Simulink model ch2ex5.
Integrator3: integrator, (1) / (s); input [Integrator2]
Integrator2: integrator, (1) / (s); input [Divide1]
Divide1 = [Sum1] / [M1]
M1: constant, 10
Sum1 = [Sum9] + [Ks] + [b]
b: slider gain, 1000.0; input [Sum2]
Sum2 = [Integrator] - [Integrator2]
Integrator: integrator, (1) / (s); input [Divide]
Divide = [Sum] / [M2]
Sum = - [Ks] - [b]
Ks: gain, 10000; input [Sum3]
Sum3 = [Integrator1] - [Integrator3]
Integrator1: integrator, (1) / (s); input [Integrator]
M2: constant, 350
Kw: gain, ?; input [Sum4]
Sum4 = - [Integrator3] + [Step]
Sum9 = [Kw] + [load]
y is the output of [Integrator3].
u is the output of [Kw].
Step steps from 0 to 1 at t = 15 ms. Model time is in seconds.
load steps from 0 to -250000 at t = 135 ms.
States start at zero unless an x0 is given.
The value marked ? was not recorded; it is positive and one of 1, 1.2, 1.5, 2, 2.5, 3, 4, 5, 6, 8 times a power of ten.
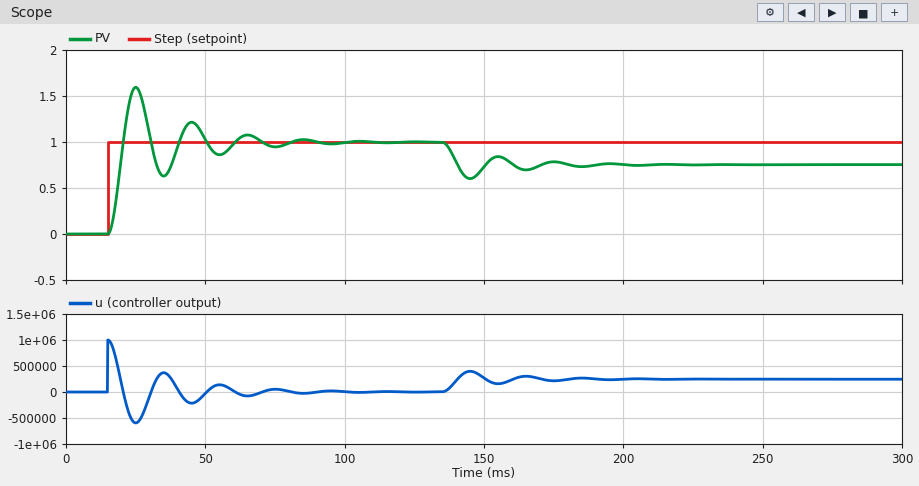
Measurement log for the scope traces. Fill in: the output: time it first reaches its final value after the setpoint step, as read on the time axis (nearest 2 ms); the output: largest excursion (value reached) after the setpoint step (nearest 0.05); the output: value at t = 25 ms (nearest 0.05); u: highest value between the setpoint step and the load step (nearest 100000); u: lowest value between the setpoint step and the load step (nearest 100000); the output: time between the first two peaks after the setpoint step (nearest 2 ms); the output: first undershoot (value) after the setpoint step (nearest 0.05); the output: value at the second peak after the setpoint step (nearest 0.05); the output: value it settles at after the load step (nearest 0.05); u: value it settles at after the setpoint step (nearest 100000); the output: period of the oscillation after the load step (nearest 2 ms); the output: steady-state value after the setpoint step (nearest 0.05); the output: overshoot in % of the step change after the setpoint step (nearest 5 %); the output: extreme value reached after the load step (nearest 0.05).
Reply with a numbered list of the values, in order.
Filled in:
1. 20 ms
2. 1.60
3. 1.60
4. 1000000
5. -600000
6. 20 ms
7. 0.65
8. 1.20
9. 0.75
10. 0
11. 20 ms
12. 1.00
13. 60 %
14. 0.60
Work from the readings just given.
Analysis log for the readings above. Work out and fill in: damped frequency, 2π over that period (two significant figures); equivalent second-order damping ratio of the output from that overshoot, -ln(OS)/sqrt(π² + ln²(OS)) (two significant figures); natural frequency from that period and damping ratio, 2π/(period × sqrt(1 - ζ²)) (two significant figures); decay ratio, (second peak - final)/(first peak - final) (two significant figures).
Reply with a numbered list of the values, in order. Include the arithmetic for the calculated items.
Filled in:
1. 2π / 20 = 0.31 rad/ms
2. ln(0.6) = -0.511; 0.511 / sqrt(9.870 + 0.261) = 0.16
3. 2π / (20 × sqrt(1 - 0.16²)) = 0.32 rad/ms
4. (1.2 - 1) / (1.6 - 1) = 0.33
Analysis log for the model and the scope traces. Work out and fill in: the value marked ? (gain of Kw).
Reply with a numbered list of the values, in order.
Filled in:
1. 1e+06
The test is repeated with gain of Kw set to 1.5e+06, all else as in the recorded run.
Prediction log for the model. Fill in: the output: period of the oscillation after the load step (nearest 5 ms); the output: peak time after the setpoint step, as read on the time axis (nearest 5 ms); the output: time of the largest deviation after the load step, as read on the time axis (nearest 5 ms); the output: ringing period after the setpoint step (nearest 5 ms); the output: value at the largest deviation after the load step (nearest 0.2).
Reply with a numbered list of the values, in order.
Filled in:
1. 15 ms
2. 25 ms
3. 145 ms
4. 15 ms
5. 0.8
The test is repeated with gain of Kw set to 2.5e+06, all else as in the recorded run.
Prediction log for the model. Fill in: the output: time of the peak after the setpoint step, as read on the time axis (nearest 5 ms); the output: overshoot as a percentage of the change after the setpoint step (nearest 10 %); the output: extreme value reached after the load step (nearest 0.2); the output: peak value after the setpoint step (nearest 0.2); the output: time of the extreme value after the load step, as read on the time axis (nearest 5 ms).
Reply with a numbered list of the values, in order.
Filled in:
1. 20 ms
2. 70 %
3. 0.8
4. 1.8
5. 140 ms
